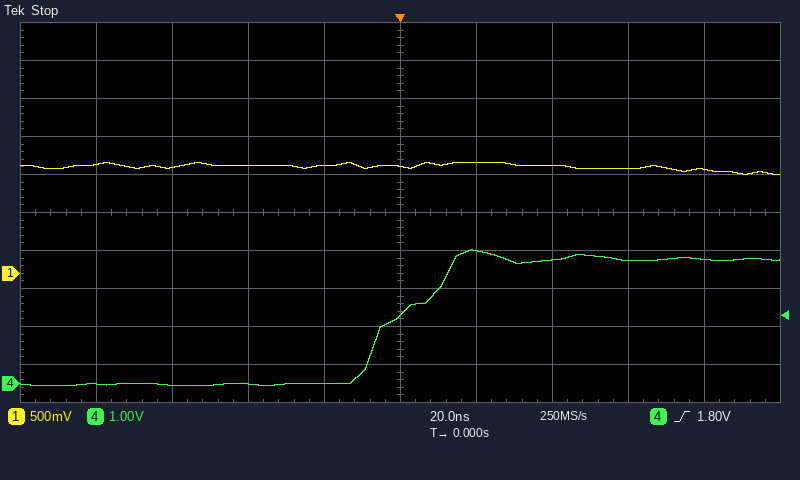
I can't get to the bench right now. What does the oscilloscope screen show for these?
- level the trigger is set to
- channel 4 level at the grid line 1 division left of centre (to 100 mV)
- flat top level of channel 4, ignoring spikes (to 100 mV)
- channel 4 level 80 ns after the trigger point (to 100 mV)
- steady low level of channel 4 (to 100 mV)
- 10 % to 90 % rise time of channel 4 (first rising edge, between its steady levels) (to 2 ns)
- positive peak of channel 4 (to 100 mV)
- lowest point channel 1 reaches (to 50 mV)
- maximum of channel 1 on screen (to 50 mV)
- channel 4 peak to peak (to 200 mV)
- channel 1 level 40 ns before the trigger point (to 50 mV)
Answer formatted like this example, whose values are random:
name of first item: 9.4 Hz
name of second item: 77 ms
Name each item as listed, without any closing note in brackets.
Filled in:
level the trigger is set to: 1.80 V
channel 4 level at the grid line 1 division left of centre: 0.0 V
flat top level of channel 4, ignoring spikes: 3.3 V
channel 4 level 80 ns after the trigger point: 3.3 V
steady low level of channel 4: 0.0 V
10 % to 90 % rise time of channel 4 (first rising edge, between its steady levels): 22 ns
positive peak of channel 4: 3.5 V
lowest point channel 1 reaches: 1.30 V
maximum of channel 1 on screen: 1.45 V
channel 4 peak to peak: 3.6 V
channel 1 level 40 ns before the trigger point: 1.40 V
